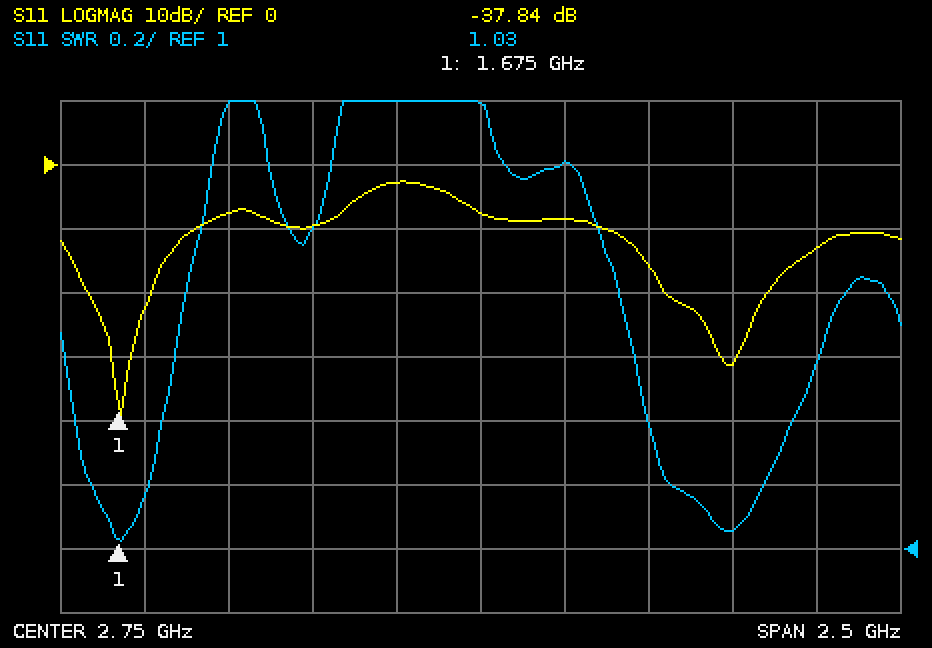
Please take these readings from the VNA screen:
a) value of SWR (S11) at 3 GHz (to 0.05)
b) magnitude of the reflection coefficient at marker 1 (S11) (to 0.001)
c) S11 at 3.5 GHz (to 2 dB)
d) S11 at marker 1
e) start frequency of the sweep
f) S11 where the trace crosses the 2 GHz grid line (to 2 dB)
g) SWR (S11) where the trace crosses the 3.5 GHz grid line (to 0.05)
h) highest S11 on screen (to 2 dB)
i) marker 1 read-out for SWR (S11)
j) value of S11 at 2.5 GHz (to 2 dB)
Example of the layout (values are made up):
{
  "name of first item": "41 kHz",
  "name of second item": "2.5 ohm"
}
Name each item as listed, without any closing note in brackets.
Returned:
{
  "value of SWR (S11) at 3 GHz": "2.20",
  "magnitude of the reflection coefficient at marker 1 (S11)": "0.013",
  "S11 at 3.5 GHz": "-32 dB",
  "S11 at marker 1": "-37.84 dB",
  "start frequency of the sweep": "1.5 GHz",
  "S11 where the trace crosses the 2 GHz grid line": "-8 dB",
  "SWR (S11) where the trace crosses the 3.5 GHz grid line": "1.05",
  "highest S11 on screen": "-2 dB",
  "marker 1 read-out for SWR": "1.03",
  "value of S11 at 2.5 GHz": "-2 dB"
}
